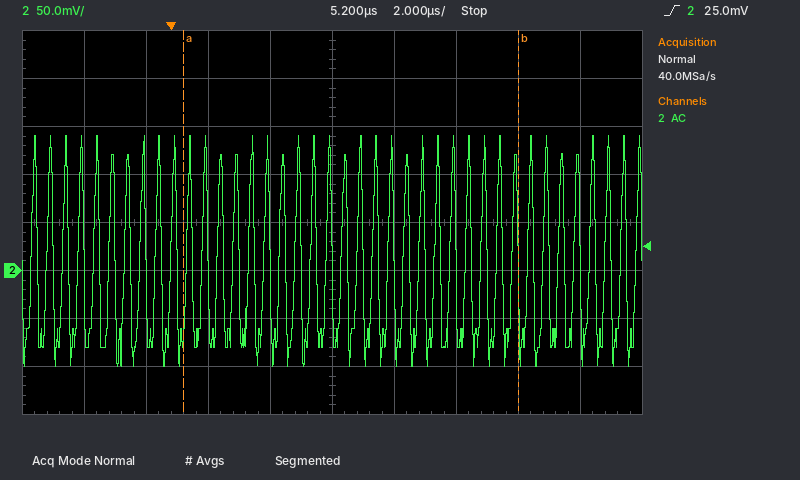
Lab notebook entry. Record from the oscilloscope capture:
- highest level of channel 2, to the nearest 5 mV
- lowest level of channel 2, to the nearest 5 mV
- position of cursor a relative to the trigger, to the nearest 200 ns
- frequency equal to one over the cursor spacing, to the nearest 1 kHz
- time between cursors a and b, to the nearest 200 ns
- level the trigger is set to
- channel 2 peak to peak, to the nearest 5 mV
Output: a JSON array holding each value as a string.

["140 mV", "-100 mV", "+400 ns", "93 kHz", "10.8 µs", "25.0 mV", "240 mV"]
